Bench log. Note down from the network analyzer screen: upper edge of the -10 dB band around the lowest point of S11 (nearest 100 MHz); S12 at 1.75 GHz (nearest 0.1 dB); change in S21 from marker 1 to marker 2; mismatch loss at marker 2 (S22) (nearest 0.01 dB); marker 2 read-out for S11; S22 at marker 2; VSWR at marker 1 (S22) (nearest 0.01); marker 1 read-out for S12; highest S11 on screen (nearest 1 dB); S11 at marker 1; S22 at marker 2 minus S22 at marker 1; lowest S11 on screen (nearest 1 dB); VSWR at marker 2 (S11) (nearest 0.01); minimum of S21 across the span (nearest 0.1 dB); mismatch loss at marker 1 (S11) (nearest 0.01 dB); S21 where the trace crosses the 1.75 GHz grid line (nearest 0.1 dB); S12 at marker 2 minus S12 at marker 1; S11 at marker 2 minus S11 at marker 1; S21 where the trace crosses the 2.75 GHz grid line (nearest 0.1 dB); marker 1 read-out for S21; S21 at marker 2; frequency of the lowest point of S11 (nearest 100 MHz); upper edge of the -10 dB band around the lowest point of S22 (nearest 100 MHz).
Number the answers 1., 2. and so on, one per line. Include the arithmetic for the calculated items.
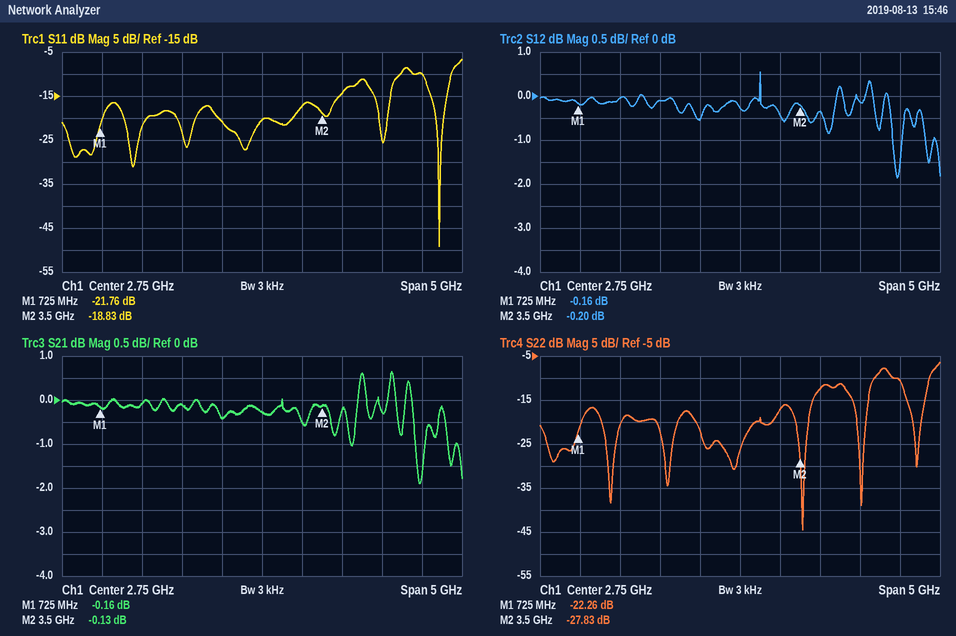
1. 5.1 GHz
2. -0.1 dB
3. -0.13 − (-0.16) = 0.03 dB
4. −10 log10(1 − 10^(-27.83/10)) ≈ 0.01 dB
5. -18.83 dB
6. -27.83 dB
7. (1 + 0.0771)/(1 − 0.0771) ≈ 1.17
8. -0.16 dB
9. -7 dB
10. -21.76 dB
11. -27.83 − (-22.26) = -5.57 dB
12. -49 dB
13. (1 + 0.1144)/(1 − 0.1144) ≈ 1.26
14. -1.9 dB
15. −10 log10(1 − 10^(-21.76/10)) ≈ 0.03 dB
16. -0.1 dB
17. -0.2 − (-0.16) = -0.04 dB
18. -18.83 − (-21.76) = 2.93 dB
19. -0.3 dB
20. -0.16 dB
21. -0.13 dB
22. 5.0 GHz
23. 4.4 GHz
